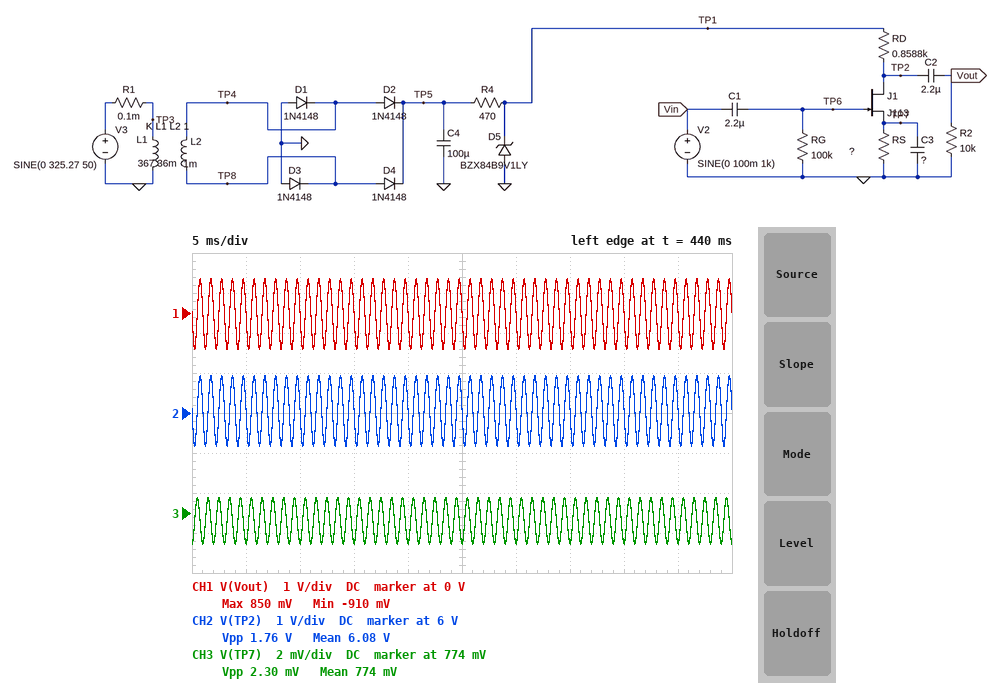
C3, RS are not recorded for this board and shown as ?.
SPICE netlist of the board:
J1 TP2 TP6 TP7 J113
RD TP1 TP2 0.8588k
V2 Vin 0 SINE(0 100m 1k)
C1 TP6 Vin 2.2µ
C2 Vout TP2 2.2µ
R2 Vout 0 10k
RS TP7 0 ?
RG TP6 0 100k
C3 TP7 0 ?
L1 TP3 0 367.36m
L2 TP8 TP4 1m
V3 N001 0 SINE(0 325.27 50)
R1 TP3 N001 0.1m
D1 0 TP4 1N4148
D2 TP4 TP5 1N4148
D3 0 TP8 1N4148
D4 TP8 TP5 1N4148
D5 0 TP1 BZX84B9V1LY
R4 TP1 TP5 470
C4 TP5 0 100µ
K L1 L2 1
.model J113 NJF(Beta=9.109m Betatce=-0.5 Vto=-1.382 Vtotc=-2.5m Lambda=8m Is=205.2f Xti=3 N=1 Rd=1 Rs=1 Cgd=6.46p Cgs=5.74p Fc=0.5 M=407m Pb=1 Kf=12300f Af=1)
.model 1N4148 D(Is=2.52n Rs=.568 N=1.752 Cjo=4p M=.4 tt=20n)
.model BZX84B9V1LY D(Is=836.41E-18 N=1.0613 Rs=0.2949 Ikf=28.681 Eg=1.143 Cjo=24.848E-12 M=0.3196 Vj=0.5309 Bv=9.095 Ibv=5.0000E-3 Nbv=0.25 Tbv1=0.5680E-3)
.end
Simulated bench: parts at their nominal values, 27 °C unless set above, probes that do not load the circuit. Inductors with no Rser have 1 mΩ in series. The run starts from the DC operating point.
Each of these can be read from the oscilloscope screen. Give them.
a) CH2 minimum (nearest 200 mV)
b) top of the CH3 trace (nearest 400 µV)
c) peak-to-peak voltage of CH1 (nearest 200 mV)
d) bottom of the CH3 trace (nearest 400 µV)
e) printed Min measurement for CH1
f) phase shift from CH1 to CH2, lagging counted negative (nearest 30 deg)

5.2 V
774.8 mV
1.8 V
772.4 mV
-910 mV
0 deg
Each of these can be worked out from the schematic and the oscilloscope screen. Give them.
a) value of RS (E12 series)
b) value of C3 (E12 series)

220 Ω
150 µF
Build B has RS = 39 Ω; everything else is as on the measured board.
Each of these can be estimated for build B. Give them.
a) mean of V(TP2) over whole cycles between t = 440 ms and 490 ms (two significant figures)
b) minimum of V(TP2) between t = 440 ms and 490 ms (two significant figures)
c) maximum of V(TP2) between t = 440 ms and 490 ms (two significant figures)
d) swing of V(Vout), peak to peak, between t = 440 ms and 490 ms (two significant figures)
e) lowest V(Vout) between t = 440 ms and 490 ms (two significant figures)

1.4 V
1.0 V
2.2 V
1.2 V
-410 mV
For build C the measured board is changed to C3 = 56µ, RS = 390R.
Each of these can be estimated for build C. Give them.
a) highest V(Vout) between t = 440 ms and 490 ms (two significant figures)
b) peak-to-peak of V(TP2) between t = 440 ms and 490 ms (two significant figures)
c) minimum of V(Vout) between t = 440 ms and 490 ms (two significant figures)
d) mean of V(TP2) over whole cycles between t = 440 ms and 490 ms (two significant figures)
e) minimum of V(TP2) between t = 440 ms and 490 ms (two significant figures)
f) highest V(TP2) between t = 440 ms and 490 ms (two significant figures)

680 mV
1.4 V
-750 mV
7.1 V
6.4 V
7.8 V
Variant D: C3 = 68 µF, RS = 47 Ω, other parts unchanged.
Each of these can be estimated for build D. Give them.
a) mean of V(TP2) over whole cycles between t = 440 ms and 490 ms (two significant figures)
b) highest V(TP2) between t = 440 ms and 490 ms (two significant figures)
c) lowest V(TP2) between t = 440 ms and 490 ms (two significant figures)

1.8 V
2.9 V
1.1 V
